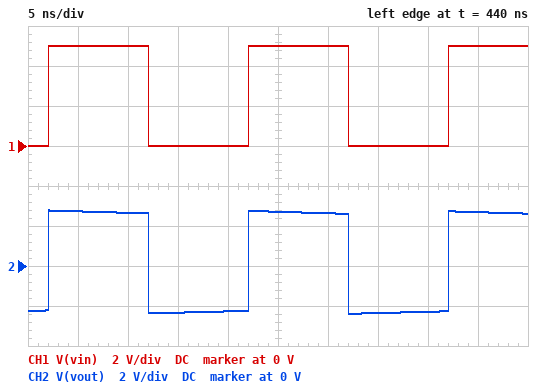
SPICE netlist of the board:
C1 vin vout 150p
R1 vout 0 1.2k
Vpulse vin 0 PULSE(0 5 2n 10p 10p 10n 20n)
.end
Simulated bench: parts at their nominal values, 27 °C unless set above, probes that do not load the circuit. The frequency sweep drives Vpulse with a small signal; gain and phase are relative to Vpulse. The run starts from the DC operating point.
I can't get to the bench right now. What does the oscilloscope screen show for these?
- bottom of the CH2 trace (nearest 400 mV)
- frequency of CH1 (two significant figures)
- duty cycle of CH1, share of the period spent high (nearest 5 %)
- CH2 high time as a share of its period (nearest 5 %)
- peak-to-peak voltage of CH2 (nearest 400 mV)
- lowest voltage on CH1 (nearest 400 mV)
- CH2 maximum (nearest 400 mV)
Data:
-2.4 V
50 MHz
50 %
50 %
5.2 V
0 V
2.8 V
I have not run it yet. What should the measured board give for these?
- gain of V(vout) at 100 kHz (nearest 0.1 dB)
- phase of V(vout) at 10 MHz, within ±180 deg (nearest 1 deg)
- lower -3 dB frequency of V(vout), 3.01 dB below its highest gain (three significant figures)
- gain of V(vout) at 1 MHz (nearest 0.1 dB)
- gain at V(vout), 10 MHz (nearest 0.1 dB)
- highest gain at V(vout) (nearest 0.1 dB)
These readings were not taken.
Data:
-19.0 dB
5 deg
884 kHz
-2.5 dB
0 dB
0 dB
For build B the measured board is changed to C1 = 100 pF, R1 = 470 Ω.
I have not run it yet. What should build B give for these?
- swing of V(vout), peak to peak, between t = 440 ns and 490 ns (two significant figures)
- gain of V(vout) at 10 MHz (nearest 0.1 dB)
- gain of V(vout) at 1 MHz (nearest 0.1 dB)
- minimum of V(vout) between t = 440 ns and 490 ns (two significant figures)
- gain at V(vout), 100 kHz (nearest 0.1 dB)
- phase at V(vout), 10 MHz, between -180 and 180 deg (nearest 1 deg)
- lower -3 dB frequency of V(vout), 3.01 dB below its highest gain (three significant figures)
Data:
5.5 V
-0.5 dB
-11.0 dB
-2.8 V
-30.6 dB
19 deg
3.39 MHz
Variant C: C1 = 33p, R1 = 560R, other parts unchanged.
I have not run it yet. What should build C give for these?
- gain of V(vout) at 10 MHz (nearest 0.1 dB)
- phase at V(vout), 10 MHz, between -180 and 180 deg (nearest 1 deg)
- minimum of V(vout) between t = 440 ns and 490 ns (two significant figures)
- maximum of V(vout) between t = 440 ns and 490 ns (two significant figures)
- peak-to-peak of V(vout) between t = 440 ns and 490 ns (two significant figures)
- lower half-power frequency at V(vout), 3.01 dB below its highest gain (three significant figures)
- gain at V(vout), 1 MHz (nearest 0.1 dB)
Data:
-2.4 dB
41 deg
-3.2 V
3.2 V
6.3 V
8.61 MHz
-18.8 dB
